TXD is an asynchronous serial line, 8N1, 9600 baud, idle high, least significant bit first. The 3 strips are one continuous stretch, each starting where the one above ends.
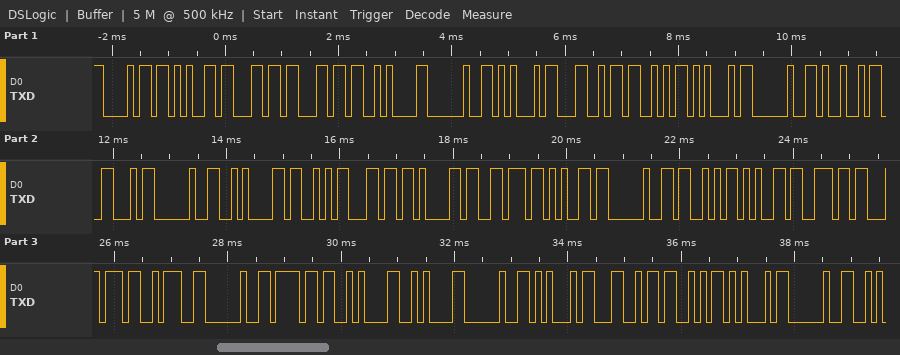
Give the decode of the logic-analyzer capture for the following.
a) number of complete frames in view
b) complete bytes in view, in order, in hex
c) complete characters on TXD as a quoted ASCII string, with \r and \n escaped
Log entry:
36
0x68 0x65 0x6C 0x6C 0x0A 0x20 0x45 0x4C 0x53 0x45 0x20 0x49 0x46 0x20 0x0A 0x53 0x6C 0x61 0x76 0x65 0x20 0x53 0x65 0x6E 0x74 0x3A 0x20 0x6F 0x0A 0x0A 0x20 0x45 0x4C 0x53 0x45 0x20
"hell\n ELSE IF \nSlave Sent: o\n\n ELSE "
